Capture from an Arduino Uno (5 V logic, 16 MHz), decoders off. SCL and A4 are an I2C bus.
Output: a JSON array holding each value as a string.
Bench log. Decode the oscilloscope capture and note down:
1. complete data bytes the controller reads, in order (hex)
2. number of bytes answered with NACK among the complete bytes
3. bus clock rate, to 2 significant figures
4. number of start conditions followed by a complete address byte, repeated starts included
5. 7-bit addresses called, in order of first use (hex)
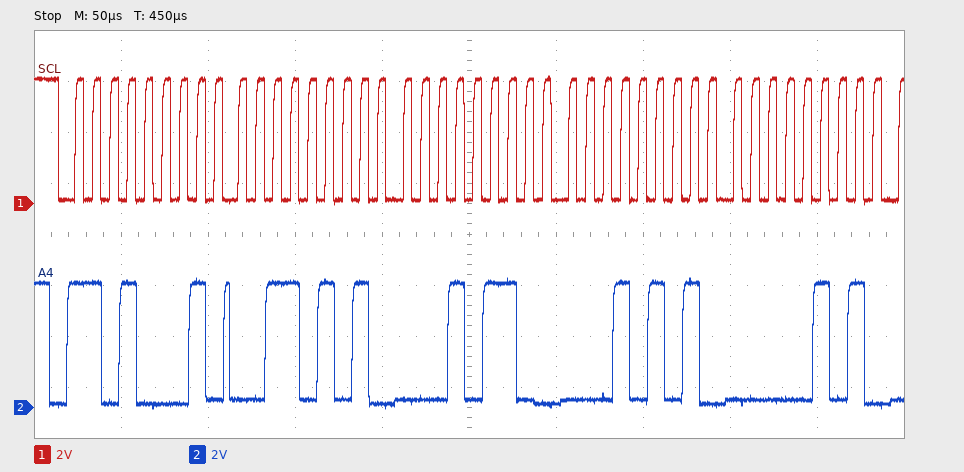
["35 16 15 05", "0", "100 kHz", "1", "0x68"]
